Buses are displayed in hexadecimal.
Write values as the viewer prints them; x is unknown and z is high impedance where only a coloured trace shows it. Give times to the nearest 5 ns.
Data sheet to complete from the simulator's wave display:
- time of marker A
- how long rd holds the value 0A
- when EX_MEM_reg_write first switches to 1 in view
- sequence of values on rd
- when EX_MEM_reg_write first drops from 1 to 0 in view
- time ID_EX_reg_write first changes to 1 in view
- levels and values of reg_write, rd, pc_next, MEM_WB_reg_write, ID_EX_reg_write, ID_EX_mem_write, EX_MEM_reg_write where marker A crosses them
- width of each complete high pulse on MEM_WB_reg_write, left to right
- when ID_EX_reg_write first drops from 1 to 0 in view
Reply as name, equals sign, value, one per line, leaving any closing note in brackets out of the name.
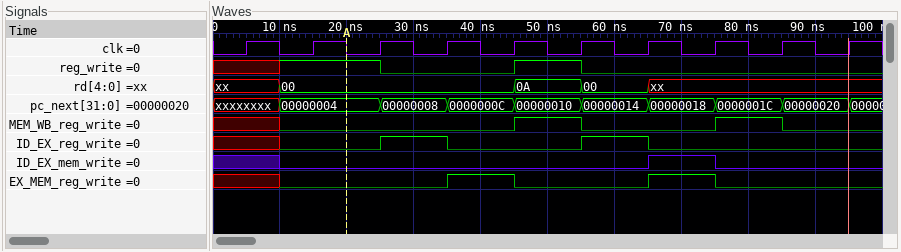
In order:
time of marker A = 20 ns
how long rd holds the value 0A = 10 ns
when EX_MEM_reg_write first switches to 1 in view = 35 ns
sequence of values on rd = xx, 00, 0A, 00, xx
when EX_MEM_reg_write first drops from 1 to 0 in view = 45 ns
time ID_EX_reg_write first changes to 1 in view = 25 ns
levels and values of reg_write, rd, pc_next, MEM_WB_reg_write, ID_EX_reg_write, ID_EX_mem_write, EX_MEM_reg_write where marker A crosses them = reg_write=1, rd=00, pc_next=00000004, MEM_WB_reg_write=0, ID_EX_reg_write=0, ID_EX_mem_write=0, EX_MEM_reg_write=0
width of each complete high pulse on MEM_WB_reg_write, left to right = 10 ns, 10 ns
when ID_EX_reg_write first drops from 1 to 0 in view = 35 ns
